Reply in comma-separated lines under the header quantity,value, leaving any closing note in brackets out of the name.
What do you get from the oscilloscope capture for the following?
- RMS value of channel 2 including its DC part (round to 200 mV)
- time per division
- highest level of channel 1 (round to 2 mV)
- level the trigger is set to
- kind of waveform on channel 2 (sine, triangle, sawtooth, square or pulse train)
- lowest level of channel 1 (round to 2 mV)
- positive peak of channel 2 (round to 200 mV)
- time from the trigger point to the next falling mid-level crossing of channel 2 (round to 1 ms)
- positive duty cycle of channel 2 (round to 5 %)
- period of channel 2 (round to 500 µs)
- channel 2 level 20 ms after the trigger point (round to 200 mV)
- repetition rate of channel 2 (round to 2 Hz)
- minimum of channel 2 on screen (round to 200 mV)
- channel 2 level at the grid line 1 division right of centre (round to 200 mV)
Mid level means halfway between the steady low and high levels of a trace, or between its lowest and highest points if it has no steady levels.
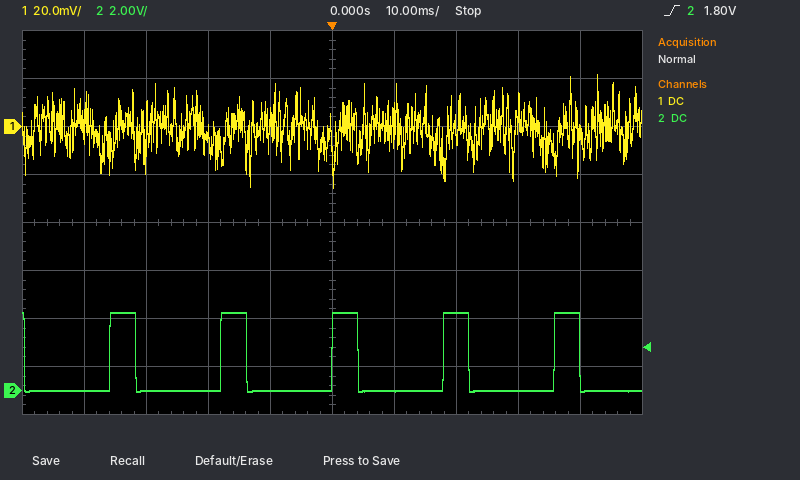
quantity,value
RMS value of channel 2 including its DC part,1.6 V
time per division,10 ms
highest level of channel 1,22 mV
level the trigger is set to,1.80 V
kind of waveform on channel 2,pulse train
lowest level of channel 1,-26 mV
positive peak of channel 2,3.2 V
time from the trigger point to the next falling mid-level crossing of channel 2,4 ms
positive duty cycle of channel 2,25 %
period of channel 2,18.0 ms
channel 2 level 20 ms after the trigger point,3.2 V
repetition rate of channel 2,56 Hz
minimum of channel 2 on screen,0.0 V
channel 2 level at the grid line 1 division right of centre,0.0 V
